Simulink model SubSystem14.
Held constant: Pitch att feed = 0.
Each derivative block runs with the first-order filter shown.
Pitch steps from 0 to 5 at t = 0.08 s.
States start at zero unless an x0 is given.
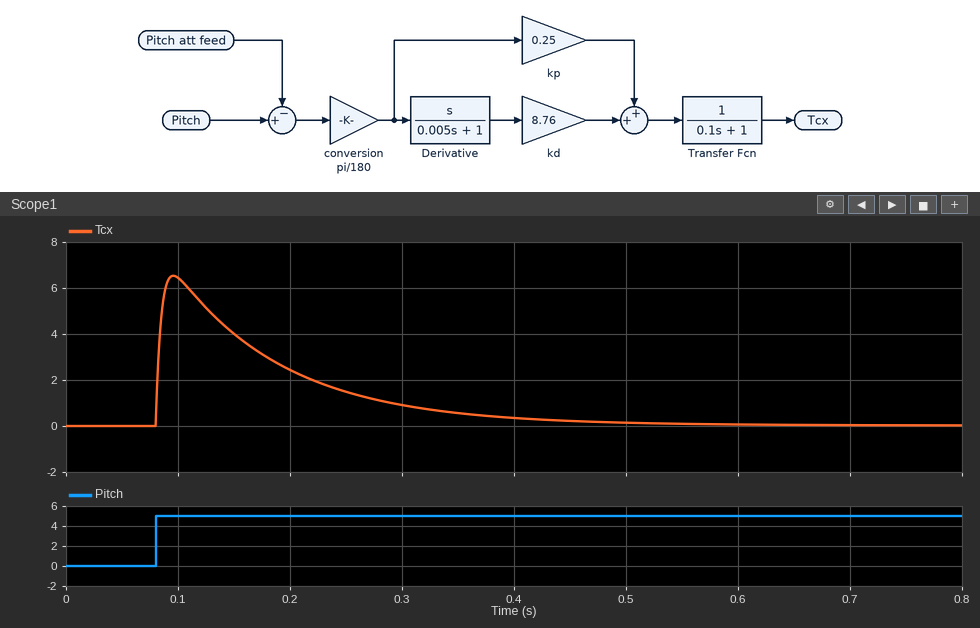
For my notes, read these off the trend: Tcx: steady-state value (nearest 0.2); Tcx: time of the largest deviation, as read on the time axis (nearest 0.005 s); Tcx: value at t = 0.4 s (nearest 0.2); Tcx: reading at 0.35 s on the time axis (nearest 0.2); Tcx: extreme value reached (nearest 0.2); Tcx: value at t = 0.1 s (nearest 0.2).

0.0
0.095 s
0.4
0.6
6.6
6.4
